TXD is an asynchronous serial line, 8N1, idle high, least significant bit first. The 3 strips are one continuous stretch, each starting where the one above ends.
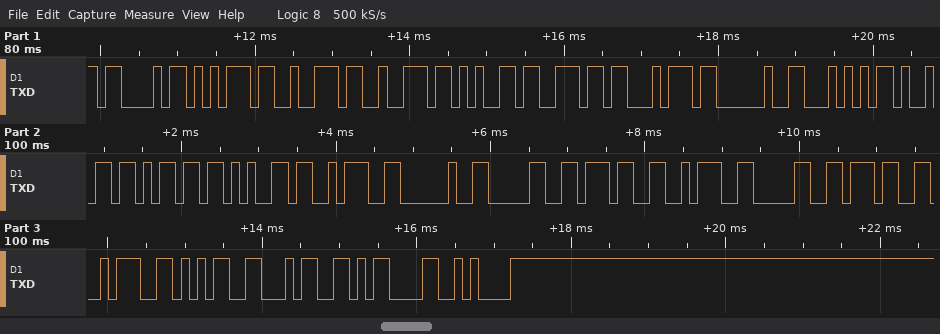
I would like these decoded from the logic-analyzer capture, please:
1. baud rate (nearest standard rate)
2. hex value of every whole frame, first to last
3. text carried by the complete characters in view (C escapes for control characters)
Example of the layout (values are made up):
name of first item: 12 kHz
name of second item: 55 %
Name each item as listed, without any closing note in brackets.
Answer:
baud rate: 9600 baud
hex value of every whole frame, first to last: 43 75 72 72 65 6E 74 20 54 69 6D 65 3A 20 30 37 3A 30 37 3A 35 34 0D 0A
text carried by the complete characters in view: "Current Time: 07:07:54\r\n"
